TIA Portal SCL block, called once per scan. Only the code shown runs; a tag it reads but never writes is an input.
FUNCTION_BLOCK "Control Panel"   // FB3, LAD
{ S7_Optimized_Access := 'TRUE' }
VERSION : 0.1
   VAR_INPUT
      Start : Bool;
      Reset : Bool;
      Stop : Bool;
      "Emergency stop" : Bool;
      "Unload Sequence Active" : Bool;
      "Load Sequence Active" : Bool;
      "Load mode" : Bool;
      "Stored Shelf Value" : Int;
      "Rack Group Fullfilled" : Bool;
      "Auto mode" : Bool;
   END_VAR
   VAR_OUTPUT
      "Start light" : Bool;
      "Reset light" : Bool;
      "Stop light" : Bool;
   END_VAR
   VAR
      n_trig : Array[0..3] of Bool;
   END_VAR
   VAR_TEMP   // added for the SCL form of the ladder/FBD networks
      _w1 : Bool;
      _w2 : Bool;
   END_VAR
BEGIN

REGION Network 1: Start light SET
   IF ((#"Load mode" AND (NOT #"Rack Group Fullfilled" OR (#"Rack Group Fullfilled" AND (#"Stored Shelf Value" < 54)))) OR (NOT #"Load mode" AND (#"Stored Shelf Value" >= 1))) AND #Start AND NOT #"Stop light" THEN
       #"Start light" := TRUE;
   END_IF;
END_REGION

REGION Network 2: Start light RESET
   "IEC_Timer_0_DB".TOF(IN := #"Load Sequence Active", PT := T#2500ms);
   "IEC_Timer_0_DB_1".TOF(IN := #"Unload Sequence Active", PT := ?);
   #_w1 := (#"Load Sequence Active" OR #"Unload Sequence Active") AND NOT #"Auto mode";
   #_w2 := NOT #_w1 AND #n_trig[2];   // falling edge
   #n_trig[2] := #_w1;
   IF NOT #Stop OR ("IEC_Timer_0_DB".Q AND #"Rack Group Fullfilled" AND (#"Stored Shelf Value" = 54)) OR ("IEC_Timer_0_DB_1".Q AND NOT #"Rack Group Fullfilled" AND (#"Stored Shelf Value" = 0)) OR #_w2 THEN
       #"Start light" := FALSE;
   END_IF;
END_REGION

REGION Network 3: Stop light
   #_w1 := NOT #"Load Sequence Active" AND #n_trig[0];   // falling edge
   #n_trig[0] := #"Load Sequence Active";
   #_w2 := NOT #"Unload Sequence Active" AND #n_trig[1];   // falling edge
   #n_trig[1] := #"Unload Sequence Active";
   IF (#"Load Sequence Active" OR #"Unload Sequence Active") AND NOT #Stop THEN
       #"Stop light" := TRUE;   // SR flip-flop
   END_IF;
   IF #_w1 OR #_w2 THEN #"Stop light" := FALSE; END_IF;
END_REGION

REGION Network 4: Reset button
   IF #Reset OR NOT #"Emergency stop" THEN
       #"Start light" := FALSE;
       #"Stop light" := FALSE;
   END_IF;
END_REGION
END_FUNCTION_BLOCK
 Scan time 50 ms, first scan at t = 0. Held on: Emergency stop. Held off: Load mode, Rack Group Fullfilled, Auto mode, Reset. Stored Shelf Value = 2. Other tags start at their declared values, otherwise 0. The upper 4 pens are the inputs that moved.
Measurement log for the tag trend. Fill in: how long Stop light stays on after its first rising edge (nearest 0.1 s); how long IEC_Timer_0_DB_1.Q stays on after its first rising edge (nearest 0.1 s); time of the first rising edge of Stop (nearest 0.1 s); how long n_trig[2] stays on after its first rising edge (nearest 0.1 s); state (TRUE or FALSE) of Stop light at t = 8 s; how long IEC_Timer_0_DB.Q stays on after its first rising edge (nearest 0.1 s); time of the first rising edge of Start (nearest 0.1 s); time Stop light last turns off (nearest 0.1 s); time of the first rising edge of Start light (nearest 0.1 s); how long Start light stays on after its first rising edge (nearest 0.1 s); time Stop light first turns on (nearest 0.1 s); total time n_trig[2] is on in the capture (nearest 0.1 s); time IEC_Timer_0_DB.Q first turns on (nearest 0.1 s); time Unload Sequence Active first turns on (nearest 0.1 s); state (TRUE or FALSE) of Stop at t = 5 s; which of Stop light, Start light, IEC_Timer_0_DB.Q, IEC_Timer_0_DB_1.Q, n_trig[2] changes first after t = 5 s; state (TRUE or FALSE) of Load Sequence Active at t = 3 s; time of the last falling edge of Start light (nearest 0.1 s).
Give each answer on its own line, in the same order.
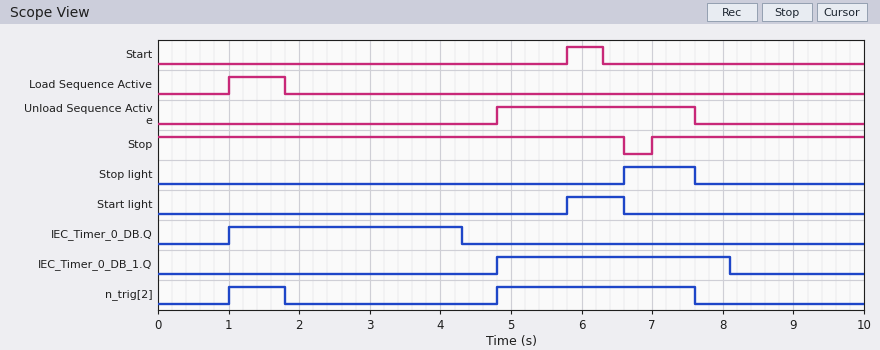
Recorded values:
1.0 s
3.3 s
7.0 s
0.8 s
FALSE
3.3 s
5.8 s
7.6 s
5.8 s
0.8 s
6.6 s
3.6 s
1.0 s
4.8 s
TRUE
Start light
FALSE
6.6 s
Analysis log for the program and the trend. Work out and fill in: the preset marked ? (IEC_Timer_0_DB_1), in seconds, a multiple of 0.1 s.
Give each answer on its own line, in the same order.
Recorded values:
0.5 s
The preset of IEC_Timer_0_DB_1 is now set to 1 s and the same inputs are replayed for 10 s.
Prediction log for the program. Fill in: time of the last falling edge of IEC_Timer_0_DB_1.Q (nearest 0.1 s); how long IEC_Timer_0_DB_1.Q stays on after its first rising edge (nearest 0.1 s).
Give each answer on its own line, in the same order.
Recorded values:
8.6 s
3.8 s
